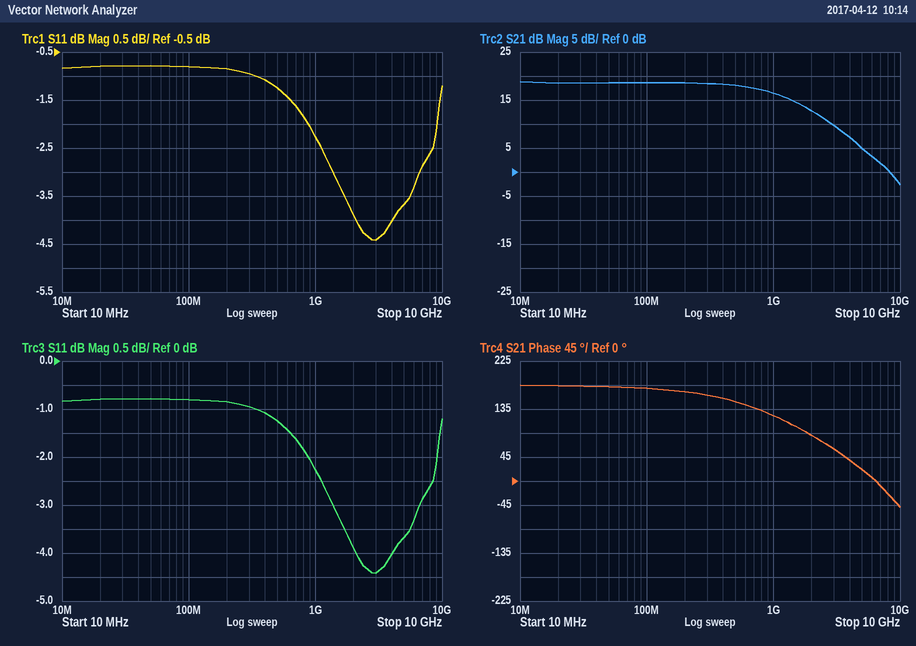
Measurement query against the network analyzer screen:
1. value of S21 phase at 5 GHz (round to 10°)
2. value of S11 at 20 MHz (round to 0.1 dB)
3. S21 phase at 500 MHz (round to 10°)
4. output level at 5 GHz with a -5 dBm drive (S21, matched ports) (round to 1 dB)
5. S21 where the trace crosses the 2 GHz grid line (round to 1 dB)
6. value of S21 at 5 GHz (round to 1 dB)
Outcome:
20°
-0.8 dB
150°
0 dBm
13 dB
5 dB
